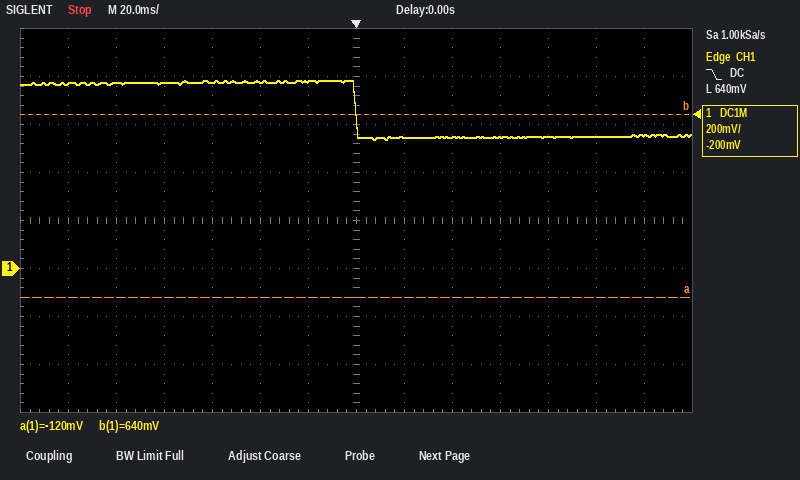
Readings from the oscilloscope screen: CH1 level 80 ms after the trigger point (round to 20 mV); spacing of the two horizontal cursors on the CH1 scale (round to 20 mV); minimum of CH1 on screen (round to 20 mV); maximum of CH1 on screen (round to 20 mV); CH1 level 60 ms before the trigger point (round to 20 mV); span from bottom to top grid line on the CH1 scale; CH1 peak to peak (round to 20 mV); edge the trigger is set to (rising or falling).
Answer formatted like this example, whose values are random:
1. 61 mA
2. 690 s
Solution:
1. 560 mV
2. 760 mV
3. 540 mV
4. 780 mV
5. 780 mV
6. 1.6 V
7. 240 mV
8. falling
